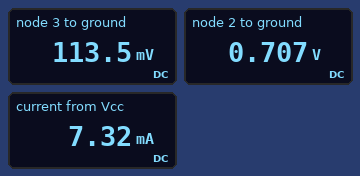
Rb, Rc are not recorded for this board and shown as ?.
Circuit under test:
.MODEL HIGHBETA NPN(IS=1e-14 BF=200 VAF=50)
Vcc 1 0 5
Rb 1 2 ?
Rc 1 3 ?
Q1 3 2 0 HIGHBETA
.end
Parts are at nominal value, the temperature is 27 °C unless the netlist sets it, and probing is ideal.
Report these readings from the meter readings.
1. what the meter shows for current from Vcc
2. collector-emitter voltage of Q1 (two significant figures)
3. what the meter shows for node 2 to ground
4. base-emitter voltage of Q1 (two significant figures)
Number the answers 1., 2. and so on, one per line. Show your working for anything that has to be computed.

1. 7.32 mA
2. 113.5 mV = 110 mV
3. 0.707 V
4. 707 mV = 710 mV
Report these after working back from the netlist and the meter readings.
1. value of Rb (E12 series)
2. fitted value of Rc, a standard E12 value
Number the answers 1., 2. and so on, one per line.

1. 33 kΩ
2. 680 Ω
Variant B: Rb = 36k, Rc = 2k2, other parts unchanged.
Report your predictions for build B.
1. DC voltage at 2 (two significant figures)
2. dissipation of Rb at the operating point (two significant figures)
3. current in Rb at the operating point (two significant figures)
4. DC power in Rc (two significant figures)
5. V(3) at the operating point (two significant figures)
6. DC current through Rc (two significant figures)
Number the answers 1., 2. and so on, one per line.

1. 680 mV
2. 520 µW
3. 120 µA
4. 11 mW
5. 81 mV
6. 2.2 mA
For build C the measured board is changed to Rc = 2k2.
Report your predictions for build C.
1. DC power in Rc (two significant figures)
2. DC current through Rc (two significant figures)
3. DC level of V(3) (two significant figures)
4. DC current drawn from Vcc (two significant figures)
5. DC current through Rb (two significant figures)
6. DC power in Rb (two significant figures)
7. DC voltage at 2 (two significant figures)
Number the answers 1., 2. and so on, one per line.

1. 11 mW
2. 2.2 mA
3. 79 mV
4. 2.4 mA
5. 130 µA
6. 570 µW
7. 680 mV
